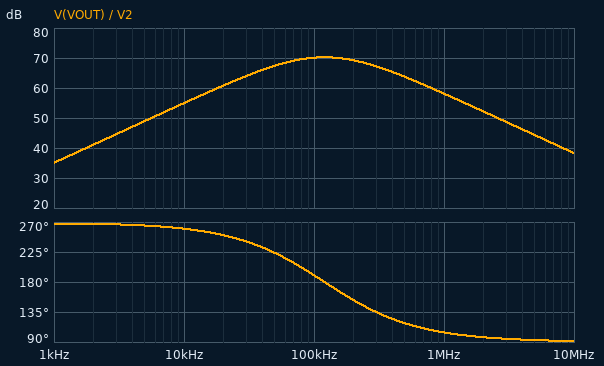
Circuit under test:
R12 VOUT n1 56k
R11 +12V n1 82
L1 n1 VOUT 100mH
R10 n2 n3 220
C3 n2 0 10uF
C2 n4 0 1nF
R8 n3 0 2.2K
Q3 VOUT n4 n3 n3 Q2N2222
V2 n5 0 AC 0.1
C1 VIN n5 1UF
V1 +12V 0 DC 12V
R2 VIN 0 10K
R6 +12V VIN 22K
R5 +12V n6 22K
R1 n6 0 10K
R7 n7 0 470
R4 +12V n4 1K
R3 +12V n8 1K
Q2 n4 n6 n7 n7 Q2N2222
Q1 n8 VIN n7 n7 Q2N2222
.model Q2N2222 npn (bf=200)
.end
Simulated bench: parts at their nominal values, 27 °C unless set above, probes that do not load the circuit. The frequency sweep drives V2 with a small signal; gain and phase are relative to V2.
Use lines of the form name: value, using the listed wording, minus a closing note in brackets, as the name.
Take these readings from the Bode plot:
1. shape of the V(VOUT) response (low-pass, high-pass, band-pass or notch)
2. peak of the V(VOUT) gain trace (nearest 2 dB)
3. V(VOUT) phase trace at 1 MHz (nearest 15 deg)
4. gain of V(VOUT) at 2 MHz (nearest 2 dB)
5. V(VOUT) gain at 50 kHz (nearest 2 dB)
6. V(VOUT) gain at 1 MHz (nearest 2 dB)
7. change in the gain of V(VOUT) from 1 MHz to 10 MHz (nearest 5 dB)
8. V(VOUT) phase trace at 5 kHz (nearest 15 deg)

shape of the V(VOUT) response: band-pass
peak of the V(VOUT) gain trace: 70 dB
V(VOUT) phase trace at 1 MHz: 105 deg
gain of V(VOUT) at 2 MHz: 52 dB
V(VOUT) gain at 50 kHz: 68 dB
V(VOUT) gain at 1 MHz: 58 dB
change in the gain of V(VOUT) from 1 MHz to 10 MHz: -20 dB
V(VOUT) phase trace at 5 kHz: 270 deg
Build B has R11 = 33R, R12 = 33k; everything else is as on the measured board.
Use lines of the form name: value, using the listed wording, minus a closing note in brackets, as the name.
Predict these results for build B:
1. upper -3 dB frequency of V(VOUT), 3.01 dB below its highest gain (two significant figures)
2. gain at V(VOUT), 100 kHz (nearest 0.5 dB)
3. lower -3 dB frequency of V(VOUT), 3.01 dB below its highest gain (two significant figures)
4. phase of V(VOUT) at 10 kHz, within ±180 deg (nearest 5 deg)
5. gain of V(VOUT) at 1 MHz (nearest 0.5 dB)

upper -3 dB frequency of V(VOUT), 3.01 dB below its highest gain: 250 kHz
gain at V(VOUT), 100 kHz: 67.0 dB
lower -3 dB frequency of V(VOUT), 3.01 dB below its highest gain: 34 kHz
phase of V(VOUT) at 10 kHz, within ±180 deg: -105 deg
gain of V(VOUT) at 1 MHz: 53.5 dB
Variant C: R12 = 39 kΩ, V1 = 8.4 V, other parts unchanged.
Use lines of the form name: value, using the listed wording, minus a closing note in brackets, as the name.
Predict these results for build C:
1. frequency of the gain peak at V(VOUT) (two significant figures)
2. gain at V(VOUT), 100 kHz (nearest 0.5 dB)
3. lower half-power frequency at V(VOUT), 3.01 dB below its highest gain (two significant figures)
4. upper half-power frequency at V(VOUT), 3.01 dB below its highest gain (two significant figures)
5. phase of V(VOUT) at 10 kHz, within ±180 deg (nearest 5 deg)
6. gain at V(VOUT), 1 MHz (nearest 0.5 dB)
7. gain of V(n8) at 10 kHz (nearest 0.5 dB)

frequency of the gain peak at V(VOUT): 100 kHz
gain at V(VOUT), 100 kHz: 66.5 dB
lower half-power frequency at V(VOUT), 3.01 dB below its highest gain: 38 kHz
upper half-power frequency at V(VOUT), 3.01 dB below its highest gain: 260 kHz
phase of V(VOUT) at 10 kHz, within ±180 deg: -105 deg
gain at V(VOUT), 1 MHz: 53.0 dB
gain of V(n8) at 10 kHz: 25.0 dB
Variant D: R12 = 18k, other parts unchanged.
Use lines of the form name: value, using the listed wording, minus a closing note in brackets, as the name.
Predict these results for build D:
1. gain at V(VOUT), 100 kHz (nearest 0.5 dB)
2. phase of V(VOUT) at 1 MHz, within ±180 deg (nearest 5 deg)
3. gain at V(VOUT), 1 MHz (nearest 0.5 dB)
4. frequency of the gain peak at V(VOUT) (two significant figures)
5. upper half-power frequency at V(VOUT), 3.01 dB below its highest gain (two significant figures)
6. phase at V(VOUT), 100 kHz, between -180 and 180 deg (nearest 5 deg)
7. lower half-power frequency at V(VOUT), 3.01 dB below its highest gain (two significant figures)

gain at V(VOUT), 100 kHz: 62.5 dB
phase of V(VOUT) at 1 MHz, within ±180 deg: 100 deg
gain at V(VOUT), 1 MHz: 48.5 dB
frequency of the gain peak at V(VOUT): 68 kHz
upper half-power frequency at V(VOUT), 3.01 dB below its highest gain: 210 kHz
phase at V(VOUT), 100 kHz, between -180 and 180 deg: 165 deg
lower half-power frequency at V(VOUT), 3.01 dB below its highest gain: 22 kHz
